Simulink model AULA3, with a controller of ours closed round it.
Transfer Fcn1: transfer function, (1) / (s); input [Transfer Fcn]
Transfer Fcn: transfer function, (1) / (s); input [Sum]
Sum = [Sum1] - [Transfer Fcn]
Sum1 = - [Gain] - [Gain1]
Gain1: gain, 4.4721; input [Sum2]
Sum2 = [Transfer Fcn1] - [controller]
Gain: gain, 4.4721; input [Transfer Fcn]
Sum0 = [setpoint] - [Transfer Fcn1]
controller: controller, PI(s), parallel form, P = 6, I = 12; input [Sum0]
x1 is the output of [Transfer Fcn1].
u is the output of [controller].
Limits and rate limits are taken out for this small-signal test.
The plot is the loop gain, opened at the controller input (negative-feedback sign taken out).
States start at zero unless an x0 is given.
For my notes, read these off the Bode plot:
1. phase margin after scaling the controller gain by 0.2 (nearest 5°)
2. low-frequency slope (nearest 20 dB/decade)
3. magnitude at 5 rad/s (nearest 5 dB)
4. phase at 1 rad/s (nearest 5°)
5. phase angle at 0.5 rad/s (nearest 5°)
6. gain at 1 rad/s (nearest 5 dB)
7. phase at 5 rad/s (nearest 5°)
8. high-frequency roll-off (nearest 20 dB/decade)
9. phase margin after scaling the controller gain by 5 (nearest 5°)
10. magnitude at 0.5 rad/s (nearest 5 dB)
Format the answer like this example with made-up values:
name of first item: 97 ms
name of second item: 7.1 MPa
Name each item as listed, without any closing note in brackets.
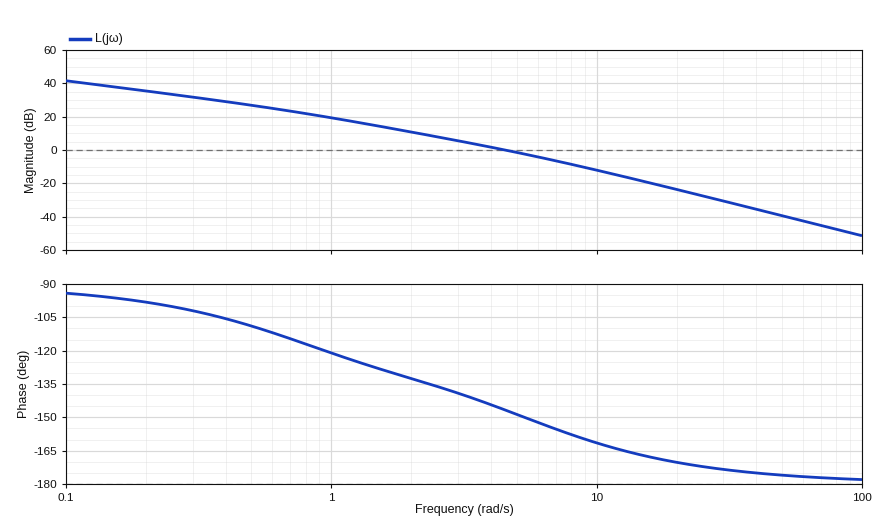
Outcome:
phase margin after scaling the controller gain by 0.2: 50°
low-frequency slope: -20 dB/decade
magnitude at 5 rad/s: 0 dB
phase at 1 rad/s: -120°
phase angle at 0.5 rad/s: -110°
gain at 1 rad/s: 20 dB
phase at 5 rad/s: -150°
high-frequency roll-off: -40 dB/decade
phase margin after scaling the controller gain by 5: 15°
magnitude at 0.5 rad/s: 25 dB
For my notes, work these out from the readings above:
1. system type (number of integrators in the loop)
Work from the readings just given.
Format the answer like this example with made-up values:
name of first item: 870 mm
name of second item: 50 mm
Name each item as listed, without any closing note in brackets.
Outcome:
system type: 1
